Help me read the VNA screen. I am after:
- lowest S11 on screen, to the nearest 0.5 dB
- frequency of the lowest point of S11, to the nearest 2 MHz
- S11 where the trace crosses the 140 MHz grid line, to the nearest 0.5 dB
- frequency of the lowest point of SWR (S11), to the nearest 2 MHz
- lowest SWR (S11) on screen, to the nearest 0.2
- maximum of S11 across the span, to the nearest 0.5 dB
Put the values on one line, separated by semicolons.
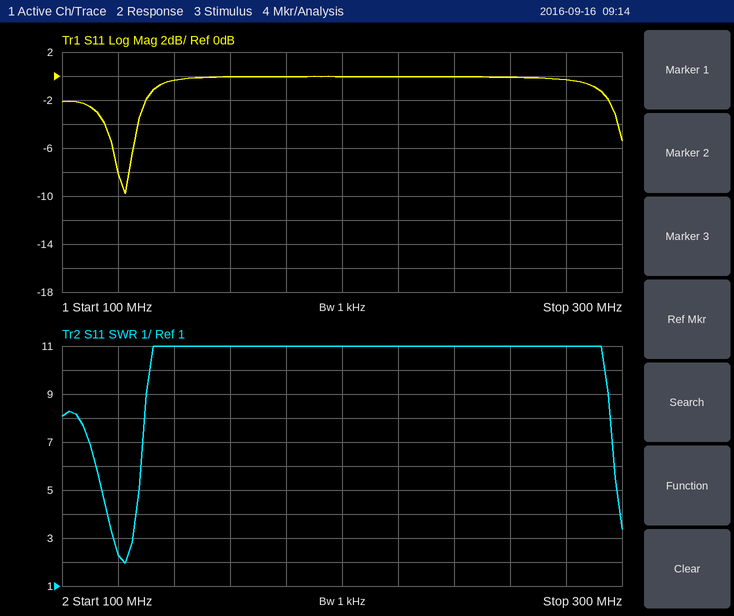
-10.0 dB; 122 MHz; -0.5 dB; 122 MHz; 2.0; 0.0 dB
